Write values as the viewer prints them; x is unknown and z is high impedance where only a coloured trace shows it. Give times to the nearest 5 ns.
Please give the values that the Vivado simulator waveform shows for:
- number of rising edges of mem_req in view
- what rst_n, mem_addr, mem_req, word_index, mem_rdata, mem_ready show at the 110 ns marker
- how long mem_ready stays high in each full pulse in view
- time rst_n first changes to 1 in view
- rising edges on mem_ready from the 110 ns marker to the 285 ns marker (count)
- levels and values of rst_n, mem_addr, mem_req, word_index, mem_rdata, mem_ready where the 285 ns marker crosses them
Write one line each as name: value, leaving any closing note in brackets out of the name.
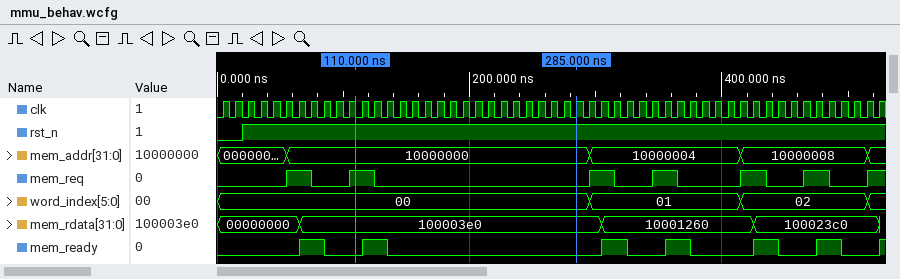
number of rising edges of mem_req in view: 7
what rst_n, mem_addr, mem_req, word_index, mem_rdata, mem_ready show at the 110 ns marker: rst_n=1, mem_addr=10000000, mem_req=1, word_index=00, mem_rdata=100003e0, mem_ready=0
how long mem_ready stays high in each full pulse in view: 20 ns, 20 ns, 20 ns, 20 ns, 20 ns, 20 ns
time rst_n first changes to 1 in view: 20 ns
rising edges on mem_ready from the 110 ns marker to the 285 ns marker: 1
levels and values of rst_n, mem_addr, mem_req, word_index, mem_rdata, mem_ready where the 285 ns marker crosses them: rst_n=1, mem_addr=10000000, mem_req=0, word_index=00, mem_rdata=100003e0, mem_ready=0
